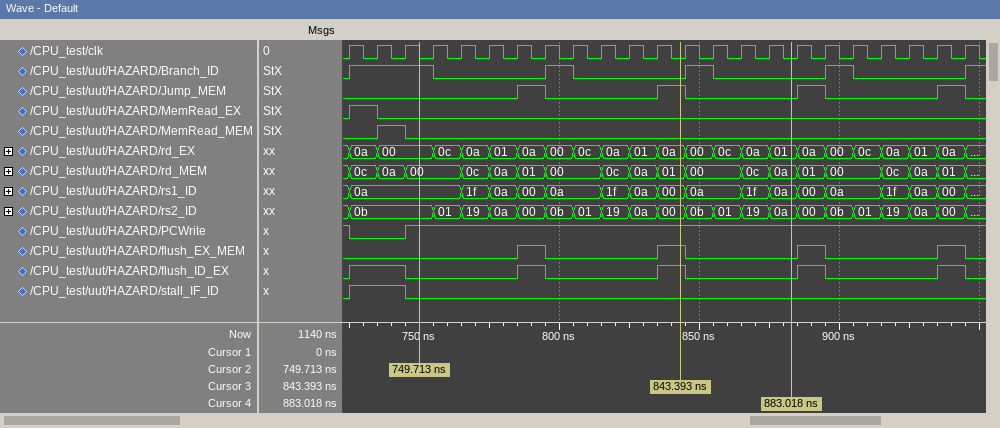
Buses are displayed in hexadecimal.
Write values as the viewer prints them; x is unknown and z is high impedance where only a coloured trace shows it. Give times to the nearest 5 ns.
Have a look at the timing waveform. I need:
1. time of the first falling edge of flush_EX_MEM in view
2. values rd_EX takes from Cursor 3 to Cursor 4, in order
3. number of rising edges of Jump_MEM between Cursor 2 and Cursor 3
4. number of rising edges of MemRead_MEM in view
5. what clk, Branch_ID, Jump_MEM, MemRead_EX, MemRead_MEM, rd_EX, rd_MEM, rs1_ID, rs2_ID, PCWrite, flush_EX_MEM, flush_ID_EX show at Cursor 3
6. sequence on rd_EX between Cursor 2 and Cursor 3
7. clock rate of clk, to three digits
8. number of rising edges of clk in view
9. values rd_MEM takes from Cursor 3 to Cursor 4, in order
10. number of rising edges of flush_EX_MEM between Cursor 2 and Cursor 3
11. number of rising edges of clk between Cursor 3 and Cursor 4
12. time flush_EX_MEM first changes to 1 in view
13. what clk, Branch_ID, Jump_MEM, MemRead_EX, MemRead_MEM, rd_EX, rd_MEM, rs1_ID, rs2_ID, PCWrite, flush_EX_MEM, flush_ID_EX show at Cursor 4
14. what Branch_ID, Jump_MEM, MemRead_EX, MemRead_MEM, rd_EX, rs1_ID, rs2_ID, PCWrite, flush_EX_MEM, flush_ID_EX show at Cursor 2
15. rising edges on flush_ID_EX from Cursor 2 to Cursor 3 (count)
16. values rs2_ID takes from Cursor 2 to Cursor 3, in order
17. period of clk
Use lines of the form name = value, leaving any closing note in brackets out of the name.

time of the first falling edge of flush_EX_MEM in view = 795 ns
values rd_EX takes from Cursor 3 to Cursor 4, in order = 0a, 00, 0c, 0a, 01
number of rising edges of Jump_MEM between Cursor 2 and Cursor 3 = 2
number of rising edges of MemRead_MEM in view = 1
what clk, Branch_ID, Jump_MEM, MemRead_EX, MemRead_MEM, rd_EX, rd_MEM, rs1_ID, rs2_ID, PCWrite, flush_EX_MEM, flush_ID_EX show at Cursor 3 = clk=0, Branch_ID=0, Jump_MEM=1, MemRead_EX=0, MemRead_MEM=0, rd_EX=0a, rd_MEM=01, rs1_ID=00, rs2_ID=00, PCWrite=1, flush_EX_MEM=1, flush_ID_EX=1
sequence on rd_EX between Cursor 2 and Cursor 3 = 00, 0c, 0a, 01, 0a, 00, 0c, 0a, 01, 0a
clock rate of clk, to three digits = 100 MHz
number of rising edges of clk in view = 23
values rd_MEM takes from Cursor 3 to Cursor 4, in order = 01, 00, 0c, 0a
number of rising edges of flush_EX_MEM between Cursor 2 and Cursor 3 = 2
number of rising edges of clk between Cursor 3 and Cursor 4 = 4
time flush_EX_MEM first changes to 1 in view = 785 ns
what clk, Branch_ID, Jump_MEM, MemRead_EX, MemRead_MEM, rd_EX, rd_MEM, rs1_ID, rs2_ID, PCWrite, flush_EX_MEM, flush_ID_EX show at Cursor 4 = clk=0, Branch_ID=0, Jump_MEM=0, MemRead_EX=0, MemRead_MEM=0, rd_EX=01, rd_MEM=0a, rs1_ID=0a, rs2_ID=0a, PCWrite=1, flush_EX_MEM=0, flush_ID_EX=0
what Branch_ID, Jump_MEM, MemRead_EX, MemRead_MEM, rd_EX, rs1_ID, rs2_ID, PCWrite, flush_EX_MEM, flush_ID_EX show at Cursor 2 = Branch_ID=1, Jump_MEM=0, MemRead_EX=0, MemRead_MEM=0, rd_EX=00, rs1_ID=0a, rs2_ID=0b, PCWrite=1, flush_EX_MEM=0, flush_ID_EX=0
rising edges on flush_ID_EX from Cursor 2 to Cursor 3 = 2
values rs2_ID takes from Cursor 2 to Cursor 3, in order = 0b, 01, 19, 0a, 00, 0b, 01, 19, 0a, 00
period of clk = 10 ns
